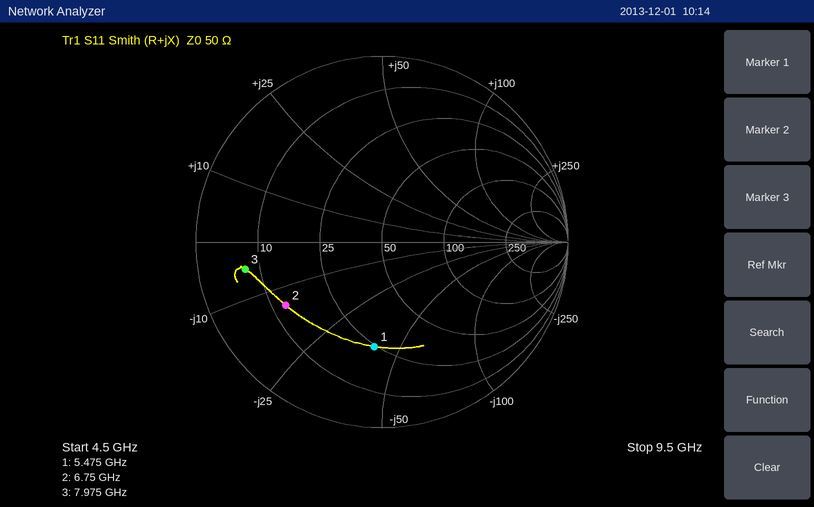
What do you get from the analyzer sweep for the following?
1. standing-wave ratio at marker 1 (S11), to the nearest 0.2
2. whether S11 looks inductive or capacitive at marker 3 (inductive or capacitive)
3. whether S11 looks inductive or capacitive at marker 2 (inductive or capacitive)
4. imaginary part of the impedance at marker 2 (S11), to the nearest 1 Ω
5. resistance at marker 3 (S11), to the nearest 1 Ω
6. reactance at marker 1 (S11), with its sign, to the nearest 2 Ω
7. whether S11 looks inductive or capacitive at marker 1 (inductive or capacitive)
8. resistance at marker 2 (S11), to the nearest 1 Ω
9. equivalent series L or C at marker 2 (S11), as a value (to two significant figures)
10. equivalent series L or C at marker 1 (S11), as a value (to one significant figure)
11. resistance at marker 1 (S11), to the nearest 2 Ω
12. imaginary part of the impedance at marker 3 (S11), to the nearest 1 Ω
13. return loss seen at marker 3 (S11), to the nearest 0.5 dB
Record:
3.6
capacitive
capacitive
-14 Ω
7 Ω
-40 Ω
capacitive
13 Ω
1.7 pF
700 fF
24 Ω
-5 Ω
2.5 dB
